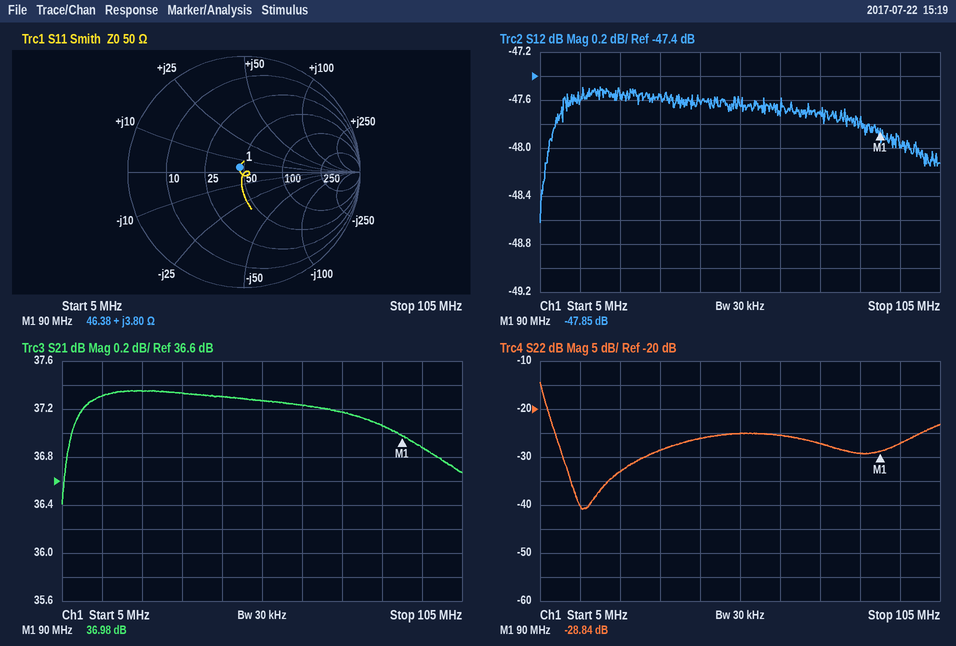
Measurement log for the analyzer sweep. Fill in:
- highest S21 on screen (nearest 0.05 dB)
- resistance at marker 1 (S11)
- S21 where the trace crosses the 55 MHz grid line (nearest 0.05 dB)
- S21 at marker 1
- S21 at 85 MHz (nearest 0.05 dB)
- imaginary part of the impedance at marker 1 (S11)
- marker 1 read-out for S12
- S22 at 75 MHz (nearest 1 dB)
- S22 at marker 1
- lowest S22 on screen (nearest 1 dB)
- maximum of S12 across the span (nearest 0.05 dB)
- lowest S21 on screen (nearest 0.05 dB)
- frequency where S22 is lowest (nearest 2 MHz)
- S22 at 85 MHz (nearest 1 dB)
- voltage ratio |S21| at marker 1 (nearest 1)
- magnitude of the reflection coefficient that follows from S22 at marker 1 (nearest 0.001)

37.35 dB
46.38 Ω
37.25 dB
36.98 dB
37.05 dB
+3.80 Ω
-47.85 dB
-27 dB
-28.84 dB
-41 dB
-47.50 dB
36.40 dB
16 MHz
-29 dB
71
0.036
